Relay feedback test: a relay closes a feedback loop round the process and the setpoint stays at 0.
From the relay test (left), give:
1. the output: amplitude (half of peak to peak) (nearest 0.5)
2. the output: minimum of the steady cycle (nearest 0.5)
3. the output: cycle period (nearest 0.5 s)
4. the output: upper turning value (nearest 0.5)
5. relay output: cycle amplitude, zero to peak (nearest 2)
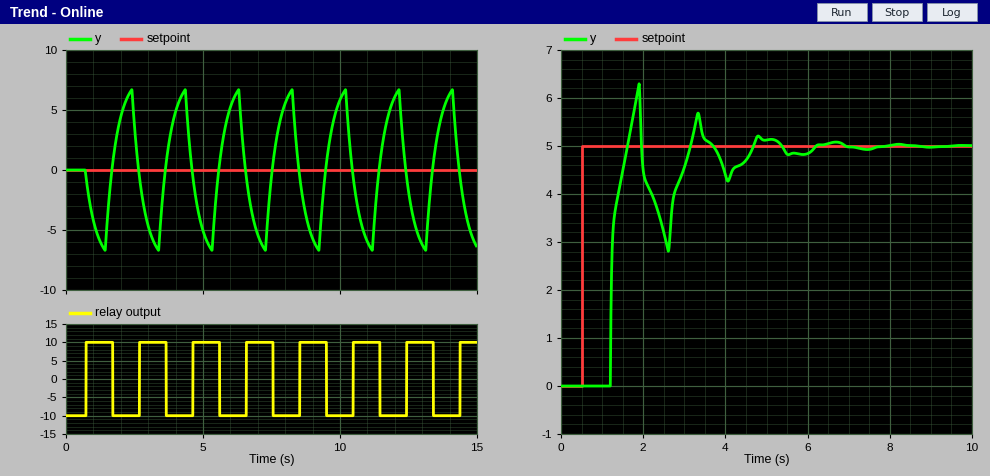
6.5
-6.5
2.0 s
6.5
10
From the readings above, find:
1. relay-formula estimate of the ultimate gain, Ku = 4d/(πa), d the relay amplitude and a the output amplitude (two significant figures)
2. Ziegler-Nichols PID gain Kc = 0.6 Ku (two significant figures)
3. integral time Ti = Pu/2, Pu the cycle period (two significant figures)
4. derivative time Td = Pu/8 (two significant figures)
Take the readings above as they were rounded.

2.0
1.2
1.0 s
0.25 s
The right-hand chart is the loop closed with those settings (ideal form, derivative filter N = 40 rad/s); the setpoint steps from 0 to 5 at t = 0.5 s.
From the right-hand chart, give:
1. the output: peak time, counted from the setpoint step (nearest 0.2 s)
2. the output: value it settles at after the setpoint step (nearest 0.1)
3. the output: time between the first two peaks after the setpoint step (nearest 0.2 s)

1.4 s
5.0
1.4 s
